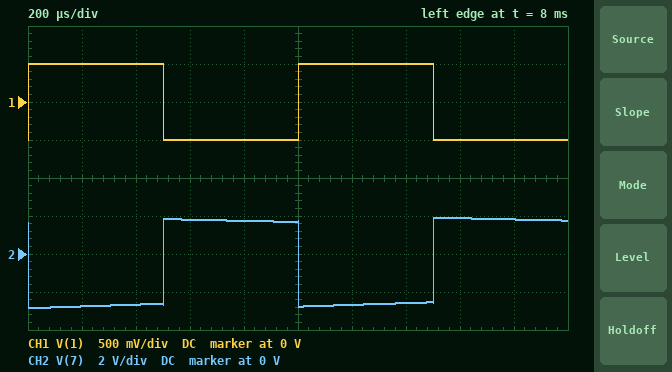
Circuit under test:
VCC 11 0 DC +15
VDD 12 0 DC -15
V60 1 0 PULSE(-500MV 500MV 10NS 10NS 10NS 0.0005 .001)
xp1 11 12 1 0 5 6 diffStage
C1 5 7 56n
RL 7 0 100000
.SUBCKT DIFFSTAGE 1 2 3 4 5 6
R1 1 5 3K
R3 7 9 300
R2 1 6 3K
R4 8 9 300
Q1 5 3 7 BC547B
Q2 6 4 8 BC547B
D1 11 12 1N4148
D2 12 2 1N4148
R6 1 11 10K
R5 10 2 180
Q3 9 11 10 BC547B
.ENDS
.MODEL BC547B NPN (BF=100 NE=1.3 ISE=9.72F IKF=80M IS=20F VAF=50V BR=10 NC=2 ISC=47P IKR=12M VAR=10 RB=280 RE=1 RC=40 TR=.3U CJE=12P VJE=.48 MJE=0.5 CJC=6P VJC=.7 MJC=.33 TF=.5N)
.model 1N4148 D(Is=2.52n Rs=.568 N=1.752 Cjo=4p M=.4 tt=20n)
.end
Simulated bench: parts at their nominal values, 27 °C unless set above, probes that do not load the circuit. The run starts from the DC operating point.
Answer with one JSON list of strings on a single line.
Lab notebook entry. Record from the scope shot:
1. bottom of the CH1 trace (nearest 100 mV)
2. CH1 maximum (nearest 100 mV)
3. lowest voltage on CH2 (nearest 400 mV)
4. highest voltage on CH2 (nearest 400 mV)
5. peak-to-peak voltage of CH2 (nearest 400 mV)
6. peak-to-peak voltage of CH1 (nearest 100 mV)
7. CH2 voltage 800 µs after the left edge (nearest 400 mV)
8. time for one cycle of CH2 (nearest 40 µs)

["-500 mV", "500 mV", "-2.8 V", "2.0 V", "4.8 V", "1.0 V", "1.6 V", "1.00 ms"]
